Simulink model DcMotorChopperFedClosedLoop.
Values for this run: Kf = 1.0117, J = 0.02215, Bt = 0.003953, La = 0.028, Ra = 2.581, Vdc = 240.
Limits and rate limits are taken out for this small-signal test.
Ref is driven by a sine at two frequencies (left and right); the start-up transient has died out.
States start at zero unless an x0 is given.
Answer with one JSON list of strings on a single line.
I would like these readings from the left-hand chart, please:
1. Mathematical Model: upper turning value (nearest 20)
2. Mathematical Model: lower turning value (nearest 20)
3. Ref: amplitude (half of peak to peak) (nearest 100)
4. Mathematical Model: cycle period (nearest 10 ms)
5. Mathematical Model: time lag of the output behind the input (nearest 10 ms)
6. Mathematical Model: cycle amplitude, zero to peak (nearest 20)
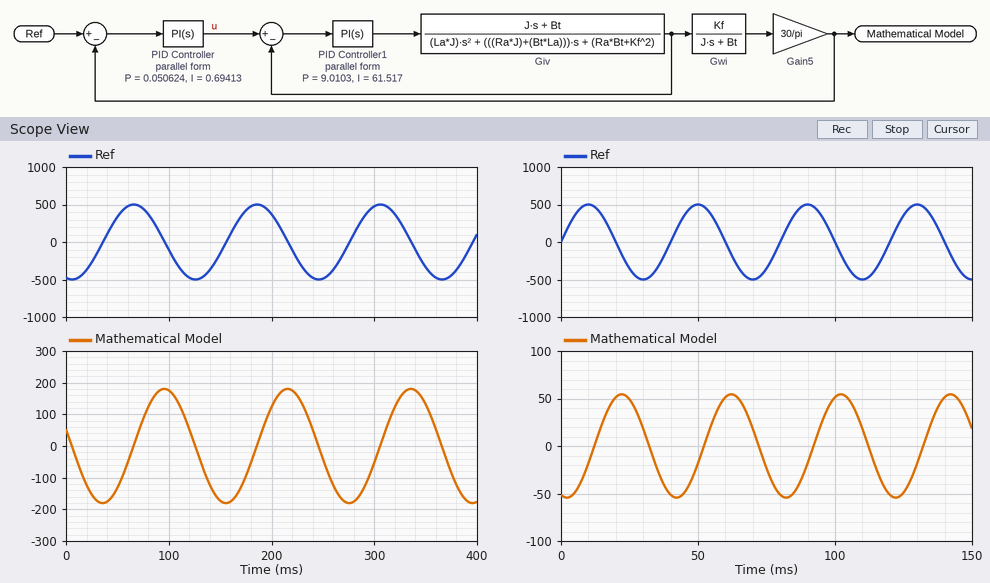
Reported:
["180", "-180", "500", "120 ms", "30 ms", "180"]
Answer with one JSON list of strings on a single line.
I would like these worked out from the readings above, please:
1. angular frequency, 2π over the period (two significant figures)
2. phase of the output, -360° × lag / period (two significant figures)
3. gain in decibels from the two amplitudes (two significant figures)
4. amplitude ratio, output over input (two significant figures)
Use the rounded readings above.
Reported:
["0.052 rad/ms", "-90°", "-8.9 dB", "0.36"]
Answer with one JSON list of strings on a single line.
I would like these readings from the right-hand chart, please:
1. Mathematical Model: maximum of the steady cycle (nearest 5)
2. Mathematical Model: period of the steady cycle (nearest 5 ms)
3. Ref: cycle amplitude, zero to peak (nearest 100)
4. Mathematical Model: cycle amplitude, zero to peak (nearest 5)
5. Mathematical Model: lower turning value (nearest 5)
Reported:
["55", "40 ms", "500", "55", "-55"]
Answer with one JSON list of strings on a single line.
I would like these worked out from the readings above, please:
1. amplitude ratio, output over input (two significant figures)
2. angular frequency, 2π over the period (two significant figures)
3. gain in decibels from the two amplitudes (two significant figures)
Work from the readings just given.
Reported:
["0.11", "0.16 rad/ms", "-19 dB"]
